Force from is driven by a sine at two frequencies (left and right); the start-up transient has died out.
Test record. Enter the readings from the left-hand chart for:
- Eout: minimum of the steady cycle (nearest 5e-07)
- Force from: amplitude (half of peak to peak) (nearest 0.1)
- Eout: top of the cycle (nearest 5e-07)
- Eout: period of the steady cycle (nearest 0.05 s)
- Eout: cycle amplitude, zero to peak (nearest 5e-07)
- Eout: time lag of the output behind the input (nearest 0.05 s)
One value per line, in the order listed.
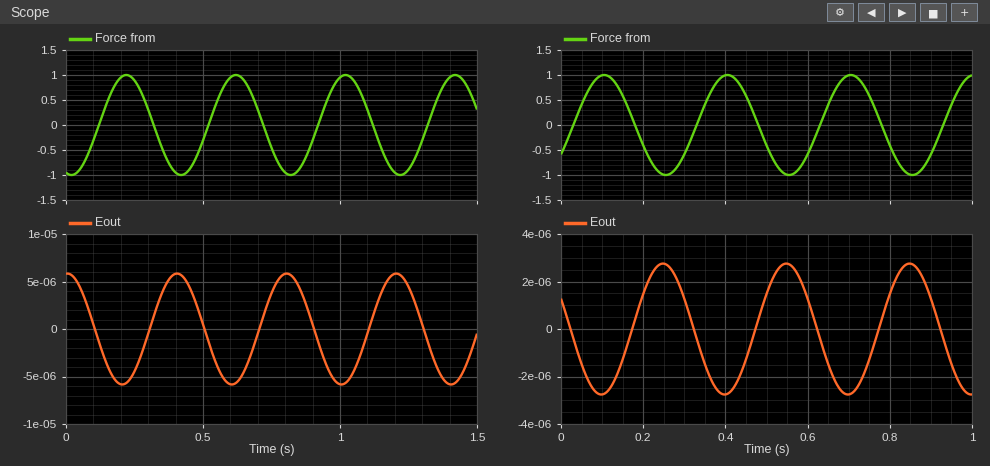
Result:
-0.0000060
1.0
0.0000060
0.40 s
0.0000060
0.20 s
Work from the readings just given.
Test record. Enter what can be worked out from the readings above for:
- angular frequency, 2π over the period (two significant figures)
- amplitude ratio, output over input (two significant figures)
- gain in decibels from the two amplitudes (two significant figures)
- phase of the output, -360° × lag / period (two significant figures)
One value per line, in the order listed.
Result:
16 rad/s
0.0000060
-100 dB
-180°
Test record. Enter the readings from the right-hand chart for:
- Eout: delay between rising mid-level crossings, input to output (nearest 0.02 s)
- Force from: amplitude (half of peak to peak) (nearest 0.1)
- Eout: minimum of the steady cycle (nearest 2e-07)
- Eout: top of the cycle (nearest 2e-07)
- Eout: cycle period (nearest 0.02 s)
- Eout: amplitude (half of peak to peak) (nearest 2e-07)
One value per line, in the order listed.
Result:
0.14 s
1.0
-0.0000028
0.0000028
0.30 s
0.0000028
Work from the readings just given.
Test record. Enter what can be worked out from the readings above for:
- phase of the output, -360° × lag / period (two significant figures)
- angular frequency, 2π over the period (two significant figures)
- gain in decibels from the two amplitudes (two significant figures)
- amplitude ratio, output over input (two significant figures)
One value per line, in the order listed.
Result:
-170°
21 rad/s
-110 dB
0.0000028
